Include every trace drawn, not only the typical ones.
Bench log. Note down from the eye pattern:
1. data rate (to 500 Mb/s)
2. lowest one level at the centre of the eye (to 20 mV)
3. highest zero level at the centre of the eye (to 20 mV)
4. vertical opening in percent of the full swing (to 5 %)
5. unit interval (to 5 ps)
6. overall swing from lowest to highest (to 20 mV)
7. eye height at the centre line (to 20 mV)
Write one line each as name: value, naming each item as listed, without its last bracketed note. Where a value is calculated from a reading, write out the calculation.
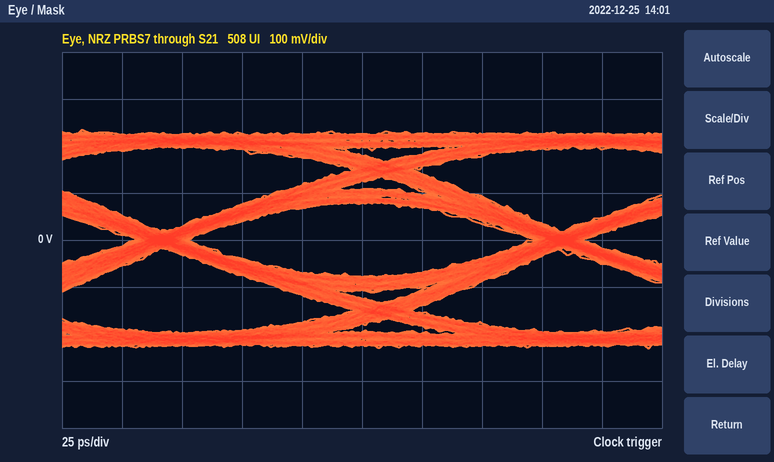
data rate: 6.0 Gb/s
lowest one level at the centre of the eye: 80 mV
highest zero level at the centre of the eye: -80 mV
vertical opening in percent of the full swing: 160 mV / 460 mV ≈ 35 %
unit interval: 165 ps
overall swing from lowest to highest: 460 mV
eye height at the centre line: 160 mV
